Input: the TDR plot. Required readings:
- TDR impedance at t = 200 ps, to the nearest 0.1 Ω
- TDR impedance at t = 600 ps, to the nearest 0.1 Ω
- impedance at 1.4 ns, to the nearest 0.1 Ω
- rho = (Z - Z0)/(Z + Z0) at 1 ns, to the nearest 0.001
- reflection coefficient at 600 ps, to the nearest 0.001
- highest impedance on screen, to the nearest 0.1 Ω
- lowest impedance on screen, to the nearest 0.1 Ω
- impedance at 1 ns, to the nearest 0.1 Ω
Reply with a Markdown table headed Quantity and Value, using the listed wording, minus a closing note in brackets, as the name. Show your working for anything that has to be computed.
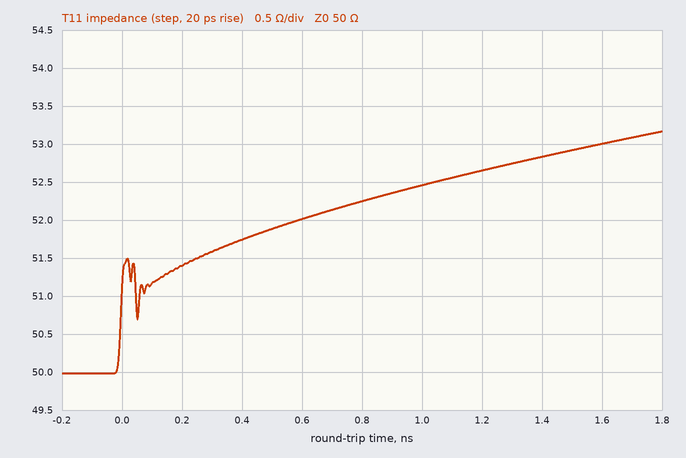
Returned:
| Quantity | Value |
|---|---|
| TDR impedance at t = 200 ps, to the nearest 0.1 Ω | 51.4 Ω |
| TDR impedance at t = 600 ps, to the nearest 0.1 Ω | 52.0 Ω |
| impedance at 1.4 ns, to the nearest 0.1 Ω | 52.8 Ω |
| rho = (Z - Z0)/(Z + Z0) at 1 ns, to the nearest 0.001 | (52.5 − 50)/(52.5 + 50) ≈ +0.024 |
| reflection coefficient at 600 ps, to the nearest 0.001 | (52 − 50)/(52 + 50) ≈ +0.020 |
| highest impedance on screen, to the nearest 0.1 Ω | 53.2 Ω |
| lowest impedance on screen, to the nearest 0.1 Ω | 50.0 Ω |
| impedance at 1 ns, to the nearest 0.1 Ω | 52.5 Ω |
